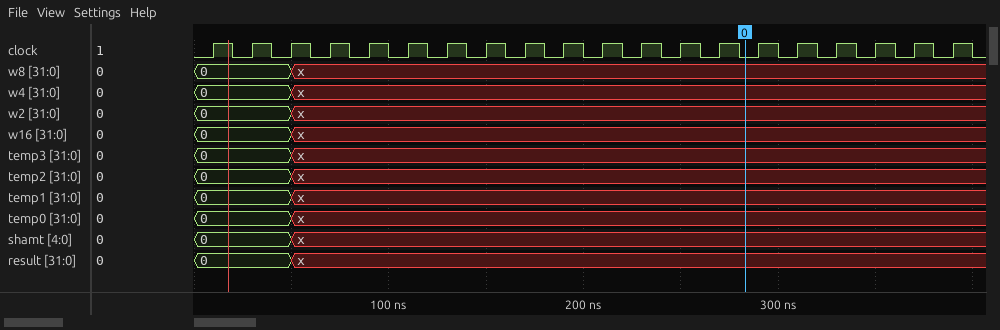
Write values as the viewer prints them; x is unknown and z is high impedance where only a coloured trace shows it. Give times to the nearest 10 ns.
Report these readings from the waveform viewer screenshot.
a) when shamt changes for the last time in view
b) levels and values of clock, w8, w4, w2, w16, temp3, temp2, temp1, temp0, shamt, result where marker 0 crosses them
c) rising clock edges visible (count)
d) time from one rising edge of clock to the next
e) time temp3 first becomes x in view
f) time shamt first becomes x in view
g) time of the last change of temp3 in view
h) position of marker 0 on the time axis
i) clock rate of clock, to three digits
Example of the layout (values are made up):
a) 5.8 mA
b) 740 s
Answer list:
a) 50 ns
b) clock=0, w8=x, w4=x, w2=x, w16=x, temp3=x, temp2=x, temp1=x, temp0=x, shamt=x, result=x
c) 20
d) 20 ns
e) 50 ns
f) 50 ns
g) 50 ns
h) 280 ns
i) 50.0 MHz
